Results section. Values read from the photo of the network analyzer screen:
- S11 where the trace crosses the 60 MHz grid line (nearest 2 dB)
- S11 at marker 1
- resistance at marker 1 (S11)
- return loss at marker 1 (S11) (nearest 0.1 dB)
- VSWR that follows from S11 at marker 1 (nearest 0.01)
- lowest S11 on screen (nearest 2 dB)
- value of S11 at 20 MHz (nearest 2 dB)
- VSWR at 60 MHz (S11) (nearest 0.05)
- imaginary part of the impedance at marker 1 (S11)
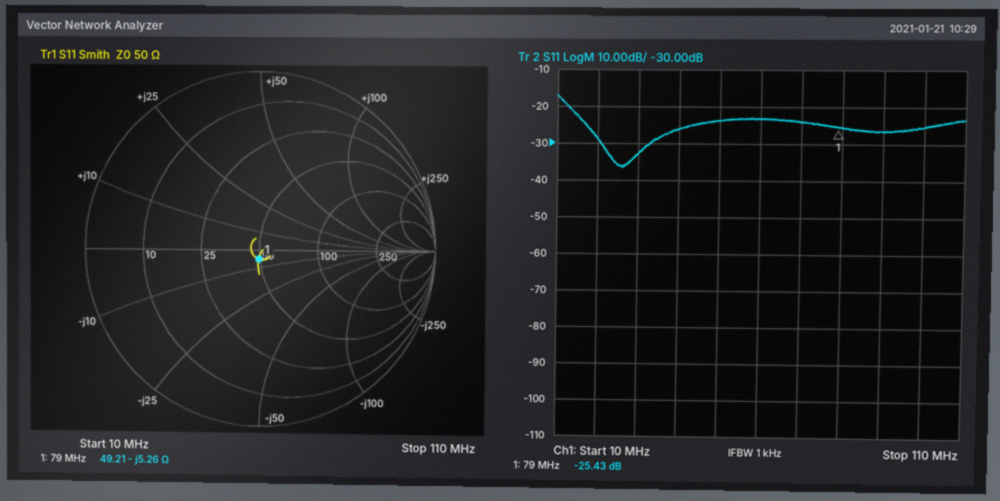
-24 dB
-25.43 dB
49.21 Ω
25.4 dB
1.11
-36 dB
-28 dB
1.15
-5.26 Ω
